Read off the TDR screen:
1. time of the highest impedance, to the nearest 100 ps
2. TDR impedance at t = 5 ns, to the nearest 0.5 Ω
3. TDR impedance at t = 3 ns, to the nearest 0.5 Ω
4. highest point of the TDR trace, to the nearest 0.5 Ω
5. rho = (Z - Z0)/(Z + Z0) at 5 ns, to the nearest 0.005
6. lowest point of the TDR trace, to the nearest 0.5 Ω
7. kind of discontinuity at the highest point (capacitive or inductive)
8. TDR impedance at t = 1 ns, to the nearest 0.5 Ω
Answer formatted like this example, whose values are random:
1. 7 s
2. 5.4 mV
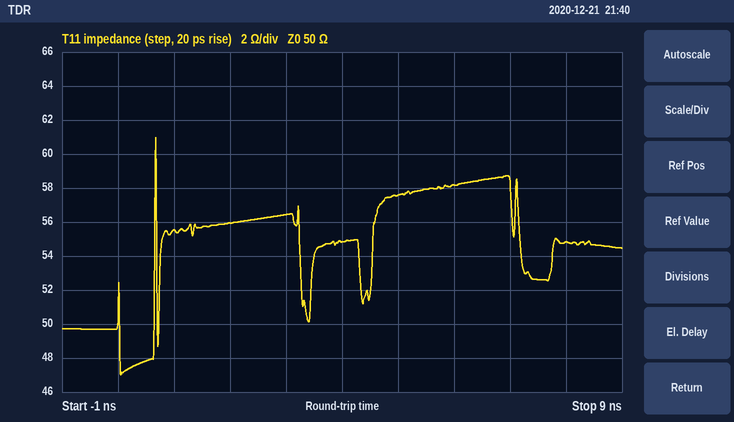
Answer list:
1. 700 ps
2. 57.5 Ω
3. 56.5 Ω
4. 61.0 Ω
5. +0.070
6. 47.0 Ω
7. inductive
8. 55.5 Ω
